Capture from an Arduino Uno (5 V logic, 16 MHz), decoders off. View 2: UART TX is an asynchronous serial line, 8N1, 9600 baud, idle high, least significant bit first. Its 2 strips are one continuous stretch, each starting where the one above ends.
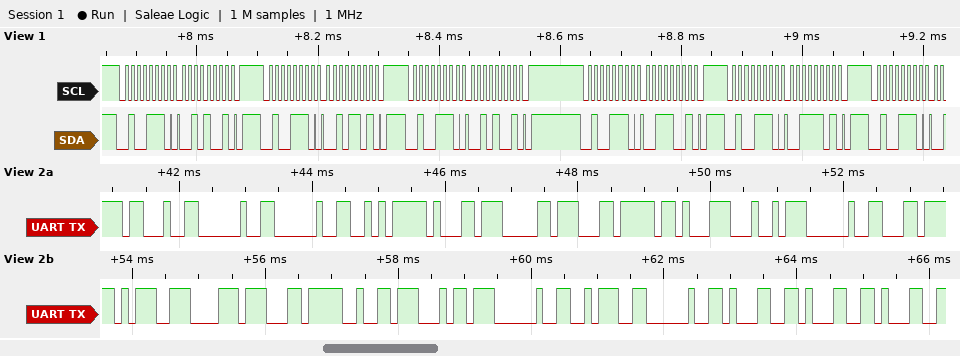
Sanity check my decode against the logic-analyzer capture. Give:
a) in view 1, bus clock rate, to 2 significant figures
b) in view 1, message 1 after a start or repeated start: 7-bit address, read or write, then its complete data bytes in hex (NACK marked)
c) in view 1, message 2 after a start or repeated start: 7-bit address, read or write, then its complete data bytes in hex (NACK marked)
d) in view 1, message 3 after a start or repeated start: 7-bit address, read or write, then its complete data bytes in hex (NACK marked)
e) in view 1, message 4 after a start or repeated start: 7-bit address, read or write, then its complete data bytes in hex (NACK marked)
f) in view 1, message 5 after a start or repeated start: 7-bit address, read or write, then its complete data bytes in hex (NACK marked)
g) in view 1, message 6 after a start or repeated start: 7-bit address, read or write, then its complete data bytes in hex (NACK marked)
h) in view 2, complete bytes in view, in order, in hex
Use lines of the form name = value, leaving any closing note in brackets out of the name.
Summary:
in view 1, bus clock rate, to 2 significant figures = 100 kHz
in view 1, message 1 after a start or repeated start: 7-bit address, read or write, then its complete data bytes in hex = 0x27 write: 29
in view 1, message 2 after a start or repeated start: 7-bit address, read or write, then its complete data bytes in hex = 0x27 write: 2D
in view 1, message 3 after a start or repeated start: 7-bit address, read or write, then its complete data bytes in hex = 0x27 write: 29
in view 1, message 4 after a start or repeated start: 7-bit address, read or write, then its complete data bytes in hex = 0x27 write: 39
in view 1, message 5 after a start or repeated start: 7-bit address, read or write, then its complete data bytes in hex = 0x27 write: 3D
in view 1, message 6 after a start or repeated start: 7-bit address, read or write, then its complete data bytes in hex = 0x27 write
in view 2, complete bytes in view, in order, in hex = 0x23 0x20 0x20 0xEA 0xB1 0xB0 0xEC 0x8B 0xA4 0x20 0xEC 0x9D 0xB8 0xEC 0xB2 0xB4 0x20 0x3A 0x20 0x31 0x31 0x31
